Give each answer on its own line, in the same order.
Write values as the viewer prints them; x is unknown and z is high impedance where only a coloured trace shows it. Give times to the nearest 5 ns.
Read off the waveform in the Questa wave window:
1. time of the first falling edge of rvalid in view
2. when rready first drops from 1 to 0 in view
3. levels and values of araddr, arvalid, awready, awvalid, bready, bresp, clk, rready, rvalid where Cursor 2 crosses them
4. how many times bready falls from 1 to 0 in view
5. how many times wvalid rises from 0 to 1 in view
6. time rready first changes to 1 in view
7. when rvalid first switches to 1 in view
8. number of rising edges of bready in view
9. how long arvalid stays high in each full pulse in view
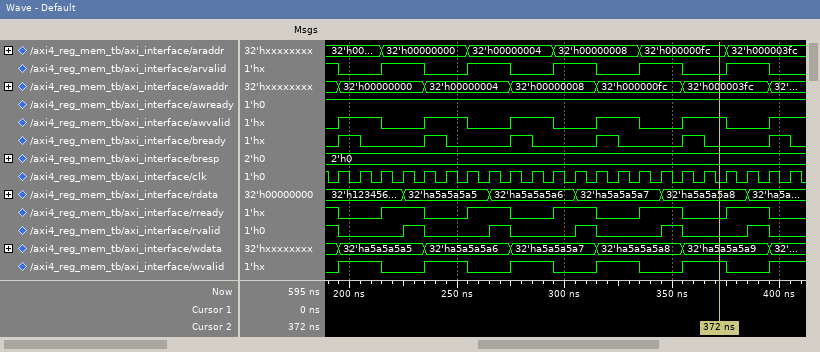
195 ns
195 ns
araddr=32'h000000fc, arvalid=0, awready=1, awvalid=1, bready=0, bresp=2'h0, clk=0, rready=0, rvalid=0
6
6
215 ns
225 ns
6
20 ns, 20 ns, 20 ns, 20 ns, 20 ns
